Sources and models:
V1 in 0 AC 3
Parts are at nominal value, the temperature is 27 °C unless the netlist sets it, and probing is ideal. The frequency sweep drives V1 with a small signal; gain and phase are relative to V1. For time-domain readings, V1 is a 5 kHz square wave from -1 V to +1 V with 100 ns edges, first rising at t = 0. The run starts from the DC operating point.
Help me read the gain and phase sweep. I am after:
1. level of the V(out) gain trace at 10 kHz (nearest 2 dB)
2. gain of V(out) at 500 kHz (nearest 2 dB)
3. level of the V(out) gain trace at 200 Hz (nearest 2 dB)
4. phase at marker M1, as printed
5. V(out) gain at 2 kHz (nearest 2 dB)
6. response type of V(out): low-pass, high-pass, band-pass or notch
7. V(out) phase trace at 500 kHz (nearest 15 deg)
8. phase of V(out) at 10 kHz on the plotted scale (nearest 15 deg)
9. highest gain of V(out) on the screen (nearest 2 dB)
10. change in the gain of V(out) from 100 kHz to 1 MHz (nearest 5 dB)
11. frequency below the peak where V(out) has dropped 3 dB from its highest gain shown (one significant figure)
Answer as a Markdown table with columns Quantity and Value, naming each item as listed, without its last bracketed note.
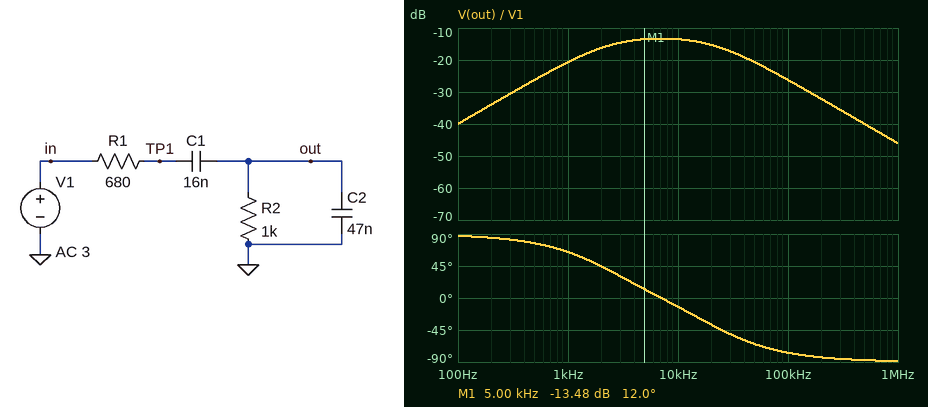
| Quantity | Value |
|---|---|
| level of the V(out) gain trace at 10 kHz | -14 dB |
| gain of V(out) at 500 kHz | -40 dB |
| level of the V(out) gain trace at 200 Hz | -34 dB |
| phase at marker M1, as printed | 12.0 deg |
| V(out) gain at 2 kHz | -16 dB |
| response type of V(out): low-pass, high-pass, band-pass or notch | band-pass |
| V(out) phase trace at 500 kHz | -90 deg |
| phase of V(out) at 10 kHz on the plotted scale | -15 deg |
| highest gain of V(out) on the screen | -14 dB |
| change in the gain of V(out) from 100 kHz to 1 MHz | -20 dB |
| frequency below the peak where V(out) has dropped 3 dB from its highest gain shown | 2 kHz |
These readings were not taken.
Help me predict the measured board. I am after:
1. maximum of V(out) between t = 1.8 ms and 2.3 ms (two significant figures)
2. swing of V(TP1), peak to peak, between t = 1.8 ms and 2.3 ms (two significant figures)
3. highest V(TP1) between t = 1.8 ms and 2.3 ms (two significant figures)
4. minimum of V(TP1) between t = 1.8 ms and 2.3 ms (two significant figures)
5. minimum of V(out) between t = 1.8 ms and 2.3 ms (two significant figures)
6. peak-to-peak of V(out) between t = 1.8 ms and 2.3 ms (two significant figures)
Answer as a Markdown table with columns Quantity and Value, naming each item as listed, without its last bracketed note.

| Quantity | Value |
|---|---|
| maximum of V(out) between t = 1.8 ms and 2.3 ms | 290 mV |
| swing of V(TP1), peak to peak, between t = 1.8 ms and 2.3 ms | 2.0 V |
| highest V(TP1) between t = 1.8 ms and 2.3 ms | 980 mV |
| minimum of V(TP1) between t = 1.8 ms and 2.3 ms | -980 mV |
| minimum of V(out) between t = 1.8 ms and 2.3 ms | -290 mV |
| peak-to-peak of V(out) between t = 1.8 ms and 2.3 ms | 580 mV |
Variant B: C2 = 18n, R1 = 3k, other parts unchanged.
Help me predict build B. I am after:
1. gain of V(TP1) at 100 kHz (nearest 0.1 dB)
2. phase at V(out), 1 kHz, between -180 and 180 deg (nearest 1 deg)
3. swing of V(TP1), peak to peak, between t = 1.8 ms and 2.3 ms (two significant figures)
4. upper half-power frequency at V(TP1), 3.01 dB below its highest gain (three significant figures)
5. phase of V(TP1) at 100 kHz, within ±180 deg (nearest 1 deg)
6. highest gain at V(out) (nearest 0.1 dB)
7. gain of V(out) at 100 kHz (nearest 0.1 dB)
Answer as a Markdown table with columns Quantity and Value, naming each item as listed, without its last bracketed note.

| Quantity | Value |
|---|---|
| gain of V(TP1) at 100 kHz | -24.1 dB |
| phase at V(out), 1 kHz, between -180 and 180 deg | 62 deg |
| swing of V(TP1), peak to peak, between t = 1.8 ms and 2.3 ms | 1.5 V |
| upper half-power frequency at V(TP1), 3.01 dB below its highest gain | 2.94 kHz |
| phase of V(TP1) at 100 kHz, within ±180 deg | -84 deg |
| highest gain at V(out) | -14.2 dB |
| gain of V(out) at 100 kHz | -30.7 dB |
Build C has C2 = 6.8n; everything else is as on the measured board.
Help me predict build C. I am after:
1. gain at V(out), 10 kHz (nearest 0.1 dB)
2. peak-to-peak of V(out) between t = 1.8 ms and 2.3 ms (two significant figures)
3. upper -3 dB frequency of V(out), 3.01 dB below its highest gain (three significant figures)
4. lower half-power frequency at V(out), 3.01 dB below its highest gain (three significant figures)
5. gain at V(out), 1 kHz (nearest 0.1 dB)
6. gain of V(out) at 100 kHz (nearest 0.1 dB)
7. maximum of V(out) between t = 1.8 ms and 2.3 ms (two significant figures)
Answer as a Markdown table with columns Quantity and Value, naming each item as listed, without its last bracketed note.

| Quantity | Value |
|---|---|
| gain at V(out), 10 kHz | -6.9 dB |
| peak-to-peak of V(out) between t = 1.8 ms and 2.3 ms | 1.6 V |
| upper -3 dB frequency of V(out), 3.01 dB below its highest gain | 76.9 kHz |
| lower half-power frequency at V(out), 3.01 dB below its highest gain | 4.45 kHz |
| gain at V(out), 1 kHz | -20.1 dB |
| gain of V(out) at 100 kHz | -10.9 dB |
| maximum of V(out) between t = 1.8 ms and 2.3 ms | 790 mV |
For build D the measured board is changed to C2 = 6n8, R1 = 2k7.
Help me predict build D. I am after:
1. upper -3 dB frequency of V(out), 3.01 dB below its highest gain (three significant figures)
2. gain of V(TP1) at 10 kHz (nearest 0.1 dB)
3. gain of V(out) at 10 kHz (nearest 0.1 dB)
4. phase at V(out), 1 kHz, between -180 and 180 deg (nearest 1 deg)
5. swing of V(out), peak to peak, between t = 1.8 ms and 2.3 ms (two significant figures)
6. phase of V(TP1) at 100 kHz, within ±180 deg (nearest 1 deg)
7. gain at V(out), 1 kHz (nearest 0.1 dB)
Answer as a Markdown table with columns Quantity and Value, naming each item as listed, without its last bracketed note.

| Quantity | Value |
|---|---|
| upper -3 dB frequency of V(out), 3.01 dB below its highest gain | 38.0 kHz |
| gain of V(TP1) at 10 kHz | -7.5 dB |
| gain of V(out) at 10 kHz | -12.3 dB |
| phase at V(out), 1 kHz, between -180 and 180 deg | 67 deg |
| swing of V(out), peak to peak, between t = 1.8 ms and 2.3 ms | 690 mV |
| phase of V(TP1) at 100 kHz, within ±180 deg | -74 deg |
| gain at V(out), 1 kHz | -20.6 dB |
